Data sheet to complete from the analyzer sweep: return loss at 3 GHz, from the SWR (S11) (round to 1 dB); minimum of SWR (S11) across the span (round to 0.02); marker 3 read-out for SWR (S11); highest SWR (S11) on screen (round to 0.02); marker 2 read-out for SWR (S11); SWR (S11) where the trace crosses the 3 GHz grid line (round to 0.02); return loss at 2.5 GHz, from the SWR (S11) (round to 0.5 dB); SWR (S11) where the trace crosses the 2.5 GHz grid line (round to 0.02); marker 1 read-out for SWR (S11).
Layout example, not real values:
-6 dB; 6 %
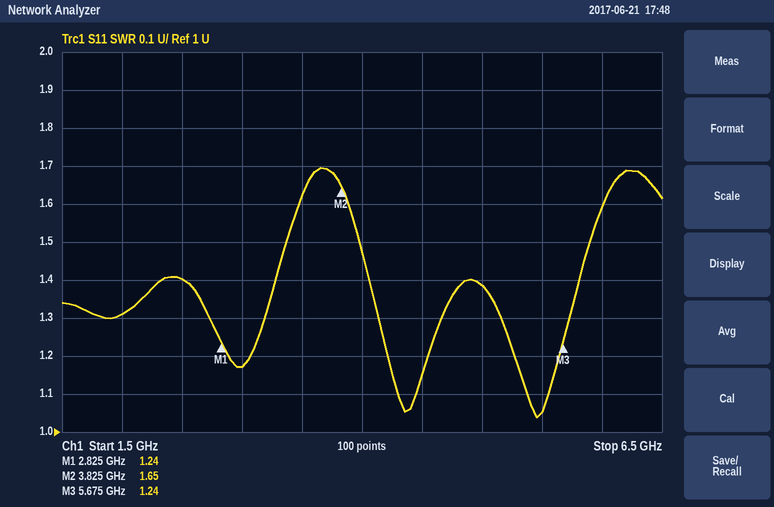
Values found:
22 dB; 1.04; 1.24; 1.70; 1.65; 1.18; 15.5 dB; 1.40; 1.24
